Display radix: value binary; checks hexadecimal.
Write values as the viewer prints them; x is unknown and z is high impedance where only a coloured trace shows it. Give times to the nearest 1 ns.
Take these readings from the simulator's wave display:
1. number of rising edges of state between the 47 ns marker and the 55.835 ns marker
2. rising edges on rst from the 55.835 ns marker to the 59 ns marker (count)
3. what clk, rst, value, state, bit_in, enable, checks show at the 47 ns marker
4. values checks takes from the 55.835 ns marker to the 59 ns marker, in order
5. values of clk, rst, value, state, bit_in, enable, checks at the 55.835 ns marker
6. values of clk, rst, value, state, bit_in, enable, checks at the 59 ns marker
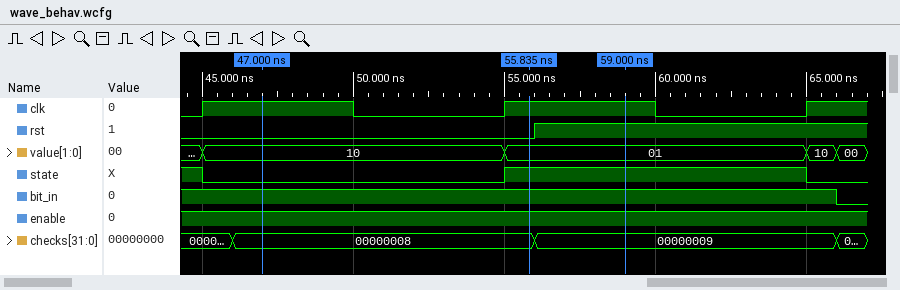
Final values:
1
1
clk=1, rst=0, value=10, state=0, bit_in=1, enable=1, checks=00000008
00000008, 00000009
clk=1, rst=0, value=01, state=1, bit_in=1, enable=1, checks=00000008
clk=1, rst=1, value=01, state=1, bit_in=1, enable=1, checks=00000009
